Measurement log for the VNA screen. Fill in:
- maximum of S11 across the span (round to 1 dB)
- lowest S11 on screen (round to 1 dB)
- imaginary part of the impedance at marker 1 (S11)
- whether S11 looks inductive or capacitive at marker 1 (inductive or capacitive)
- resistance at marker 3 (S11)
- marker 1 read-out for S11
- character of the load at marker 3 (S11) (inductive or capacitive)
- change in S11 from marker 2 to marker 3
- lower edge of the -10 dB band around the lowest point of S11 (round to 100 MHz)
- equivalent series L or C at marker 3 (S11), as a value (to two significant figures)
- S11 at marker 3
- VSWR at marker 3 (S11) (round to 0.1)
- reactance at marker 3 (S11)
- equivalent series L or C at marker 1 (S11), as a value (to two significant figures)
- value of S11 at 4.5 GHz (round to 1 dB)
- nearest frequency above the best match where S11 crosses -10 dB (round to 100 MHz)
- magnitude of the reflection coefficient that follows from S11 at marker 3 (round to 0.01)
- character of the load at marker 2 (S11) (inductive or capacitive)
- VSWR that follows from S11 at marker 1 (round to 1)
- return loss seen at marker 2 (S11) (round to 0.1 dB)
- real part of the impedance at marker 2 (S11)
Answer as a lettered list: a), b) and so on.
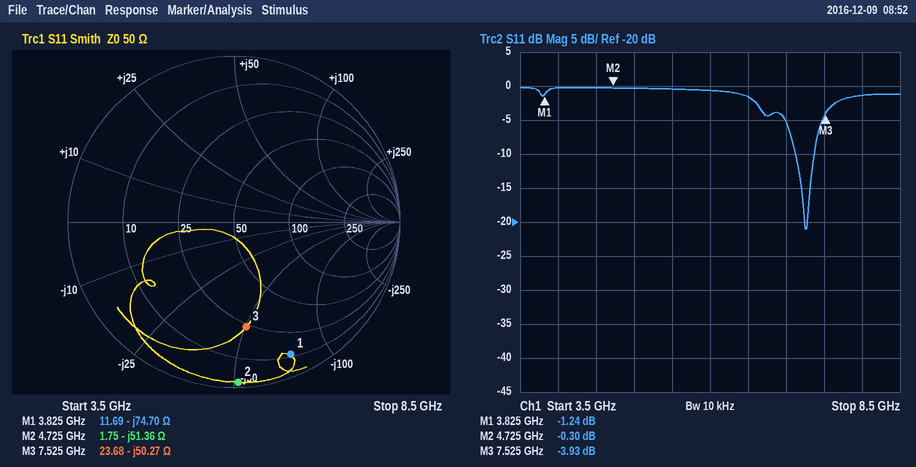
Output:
a) 0 dB
b) -21 dB
c) -74.70 Ω
d) capacitive
e) 23.68 Ω
f) -1.24 dB
g) capacitive
h) -3.63 dB
i) 7.1 GHz
j) 420 fF
k) -3.93 dB
l) 4.5
m) -50.27 Ω
n) 560 fF
o) 0 dB
p) 7.4 GHz
q) 0.64
r) capacitive
s) 14
t) 0.3 dB
u) 1.75 Ω
